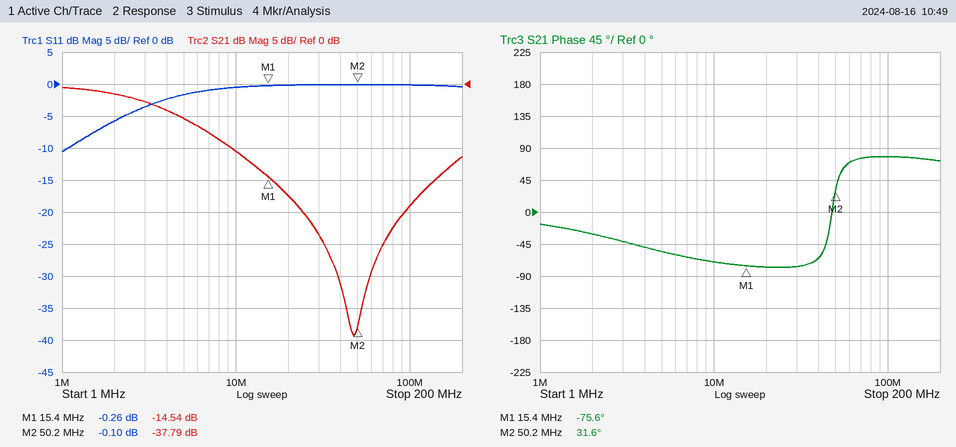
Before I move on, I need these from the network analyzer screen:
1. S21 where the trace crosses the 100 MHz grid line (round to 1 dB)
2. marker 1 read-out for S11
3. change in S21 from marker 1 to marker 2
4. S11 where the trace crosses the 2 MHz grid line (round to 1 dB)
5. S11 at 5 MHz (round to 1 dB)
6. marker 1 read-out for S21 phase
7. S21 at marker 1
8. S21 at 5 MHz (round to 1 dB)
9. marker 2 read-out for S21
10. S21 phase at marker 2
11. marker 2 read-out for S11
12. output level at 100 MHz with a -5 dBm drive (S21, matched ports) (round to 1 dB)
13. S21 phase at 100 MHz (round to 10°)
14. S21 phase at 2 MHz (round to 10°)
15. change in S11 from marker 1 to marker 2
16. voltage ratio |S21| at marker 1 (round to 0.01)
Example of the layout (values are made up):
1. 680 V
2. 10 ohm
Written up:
1. -19 dB
2. -0.26 dB
3. -23.25 dB
4. -6 dB
5. -2 dB
6. -75.6°
7. -14.54 dB
8. -5 dB
9. -37.79 dB
10. 31.6°
11. -0.10 dB
12. -24 dBm
13. 80°
14. -30°
15. 0.16 dB
16. 0.19
